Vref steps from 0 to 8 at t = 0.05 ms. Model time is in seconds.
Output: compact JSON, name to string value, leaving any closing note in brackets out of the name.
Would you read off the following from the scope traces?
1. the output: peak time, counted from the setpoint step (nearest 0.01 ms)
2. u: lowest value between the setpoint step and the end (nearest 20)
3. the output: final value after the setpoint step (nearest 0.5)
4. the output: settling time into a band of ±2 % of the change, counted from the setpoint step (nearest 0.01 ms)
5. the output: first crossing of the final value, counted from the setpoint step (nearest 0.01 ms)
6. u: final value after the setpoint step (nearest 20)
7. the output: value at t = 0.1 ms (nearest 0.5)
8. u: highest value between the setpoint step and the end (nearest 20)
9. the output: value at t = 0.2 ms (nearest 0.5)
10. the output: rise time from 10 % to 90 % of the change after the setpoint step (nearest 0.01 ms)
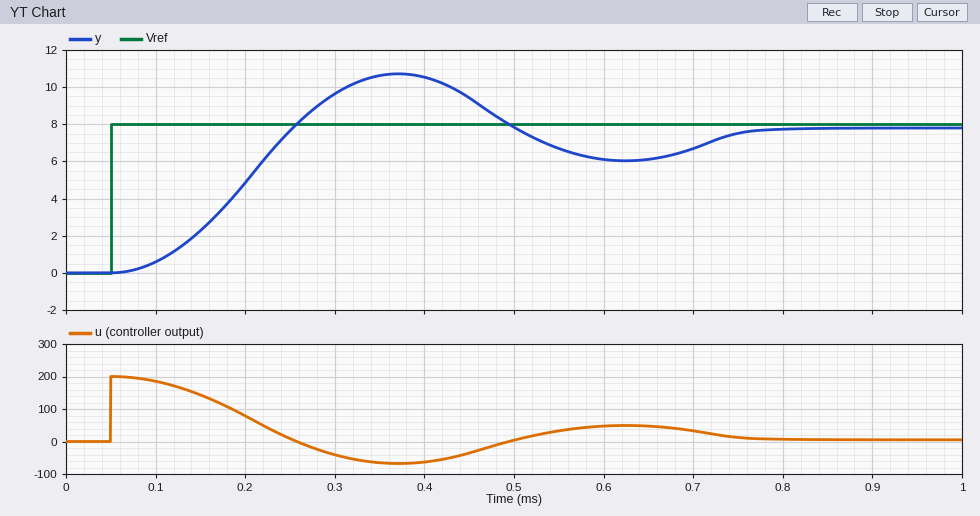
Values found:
{"the output: peak time, counted from the setpoint step": "0.32 ms", "u: lowest value between the setpoint step and the end": "-60", "the output: final value after the setpoint step": "8.0", "the output: settling time into a band of ±2 % of the change, counted from the setpoint step": "0.72 ms", "the output: first crossing of the final value, counted from the setpoint step": "0.20 ms", "u: final value after the setpoint step": "0", "the output: value at t = 0.1 ms": "0.5", "u: highest value between the setpoint step and the end": "200", "the output: value at t = 0.2 ms": "5.0", "the output: rise time from 10 % to 90 % of the change after the setpoint step": "0.13 ms"}
